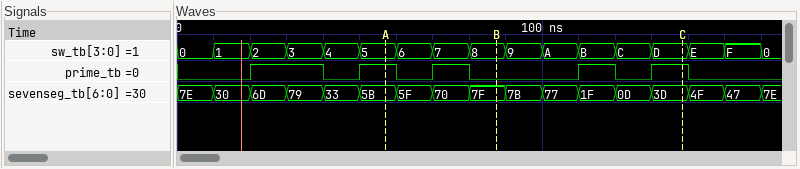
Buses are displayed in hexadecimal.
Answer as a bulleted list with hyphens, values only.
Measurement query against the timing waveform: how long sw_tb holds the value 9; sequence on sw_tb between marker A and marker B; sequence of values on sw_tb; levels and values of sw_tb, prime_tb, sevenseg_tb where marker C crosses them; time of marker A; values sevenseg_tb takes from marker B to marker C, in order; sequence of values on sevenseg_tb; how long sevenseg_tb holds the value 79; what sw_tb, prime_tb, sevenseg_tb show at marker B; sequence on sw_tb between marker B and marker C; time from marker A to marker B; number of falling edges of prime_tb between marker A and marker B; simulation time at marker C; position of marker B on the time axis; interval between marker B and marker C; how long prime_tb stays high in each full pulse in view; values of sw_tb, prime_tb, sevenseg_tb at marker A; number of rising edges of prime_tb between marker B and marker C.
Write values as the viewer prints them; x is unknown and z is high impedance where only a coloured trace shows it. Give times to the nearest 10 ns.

- 10 ns
- 5, 6, 7, 8
- 0, 1, 2, 3, 4, 5, 6, 7, 8, 9, A, B, C, D, E, F, 0
- sw_tb=D, prime_tb=1, sevenseg_tb=3D
- 60 ns
- 7F, 7B, 77, 1F, 0D, 3D
- 7E, 30, 6D, 79, 33, 5B, 5F, 70, 7F, 7B, 77, 1F, 0D, 3D, 4F, 47, 7E
- 10 ns
- sw_tb=8, prime_tb=0, sevenseg_tb=7F
- 8, 9, A, B, C, D
- 30 ns
- 2
- 140 ns
- 90 ns
- 50 ns
- 20 ns, 10 ns, 10 ns, 10 ns, 10 ns
- sw_tb=5, prime_tb=1, sevenseg_tb=5B
- 2
